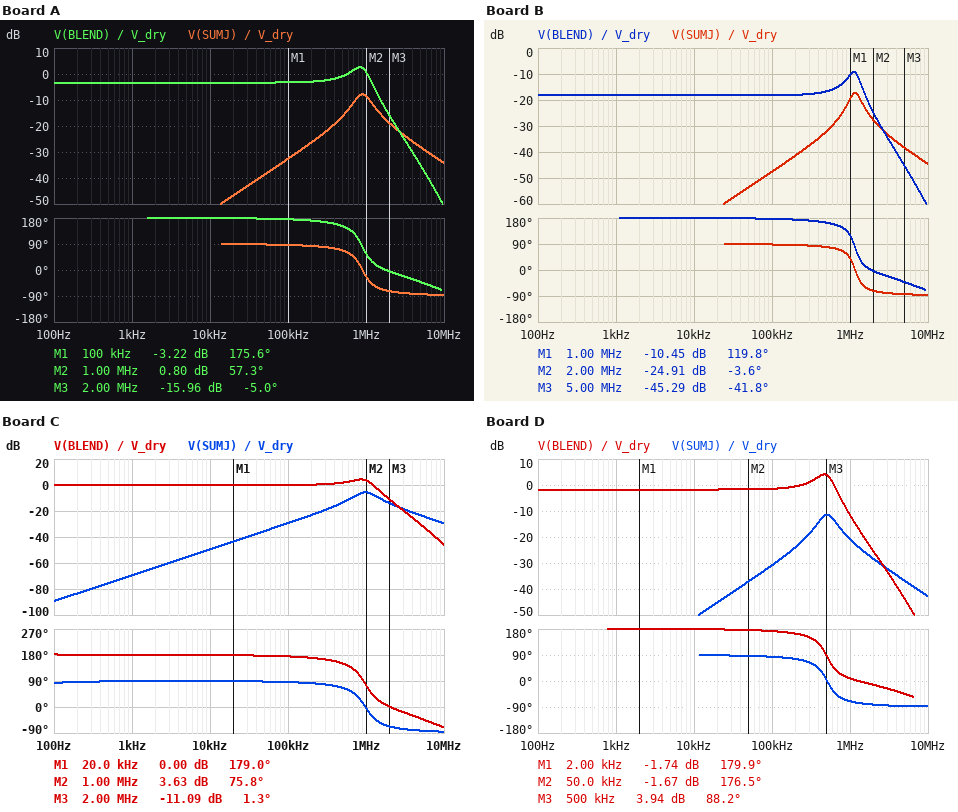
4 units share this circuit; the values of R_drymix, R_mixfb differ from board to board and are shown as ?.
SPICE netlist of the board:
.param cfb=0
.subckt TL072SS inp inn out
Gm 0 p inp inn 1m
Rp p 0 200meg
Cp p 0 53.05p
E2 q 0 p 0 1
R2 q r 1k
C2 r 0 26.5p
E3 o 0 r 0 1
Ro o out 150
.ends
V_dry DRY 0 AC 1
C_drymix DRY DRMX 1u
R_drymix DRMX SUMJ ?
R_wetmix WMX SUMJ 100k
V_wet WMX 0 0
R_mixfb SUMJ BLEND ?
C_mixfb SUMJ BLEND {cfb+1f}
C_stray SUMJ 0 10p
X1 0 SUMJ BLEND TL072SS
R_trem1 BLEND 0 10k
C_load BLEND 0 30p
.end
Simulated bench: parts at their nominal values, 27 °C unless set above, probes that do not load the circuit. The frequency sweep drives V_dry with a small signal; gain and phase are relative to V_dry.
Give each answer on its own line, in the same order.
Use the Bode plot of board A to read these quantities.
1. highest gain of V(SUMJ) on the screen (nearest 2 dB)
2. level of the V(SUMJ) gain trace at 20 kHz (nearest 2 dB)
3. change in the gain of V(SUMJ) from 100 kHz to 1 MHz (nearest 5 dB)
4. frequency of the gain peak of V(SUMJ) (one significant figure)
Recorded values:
-8 dB
-46 dB
25 dB
900 kHz
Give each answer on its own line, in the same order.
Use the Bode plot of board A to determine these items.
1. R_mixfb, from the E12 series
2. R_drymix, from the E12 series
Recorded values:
56 kΩ
82 kΩ
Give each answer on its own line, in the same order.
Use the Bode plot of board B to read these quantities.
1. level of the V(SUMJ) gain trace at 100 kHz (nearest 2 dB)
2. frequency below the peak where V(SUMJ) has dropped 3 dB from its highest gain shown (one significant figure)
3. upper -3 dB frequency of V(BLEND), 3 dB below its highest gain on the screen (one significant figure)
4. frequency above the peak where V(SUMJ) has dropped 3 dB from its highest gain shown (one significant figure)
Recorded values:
-48 dB
1 MHz
1 MHz
1 MHz
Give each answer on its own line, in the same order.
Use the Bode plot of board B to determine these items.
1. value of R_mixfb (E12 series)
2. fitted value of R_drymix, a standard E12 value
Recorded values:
33 kΩ
270 kΩ
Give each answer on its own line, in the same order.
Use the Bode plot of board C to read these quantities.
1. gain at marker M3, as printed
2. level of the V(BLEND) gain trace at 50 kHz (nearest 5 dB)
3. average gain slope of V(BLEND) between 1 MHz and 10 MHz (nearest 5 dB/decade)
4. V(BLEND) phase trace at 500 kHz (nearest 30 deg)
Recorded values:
-11.09 dB
0 dB
-50 dB/decade
150 deg
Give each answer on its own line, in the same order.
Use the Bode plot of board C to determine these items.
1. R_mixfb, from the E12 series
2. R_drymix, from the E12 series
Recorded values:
47 kΩ
47 kΩ
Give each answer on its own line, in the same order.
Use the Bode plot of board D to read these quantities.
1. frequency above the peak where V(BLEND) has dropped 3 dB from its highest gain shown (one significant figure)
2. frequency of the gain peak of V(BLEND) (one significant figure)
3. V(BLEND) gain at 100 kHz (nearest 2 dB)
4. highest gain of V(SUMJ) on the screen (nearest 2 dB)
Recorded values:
600 kHz
500 kHz
-2 dB
-12 dB
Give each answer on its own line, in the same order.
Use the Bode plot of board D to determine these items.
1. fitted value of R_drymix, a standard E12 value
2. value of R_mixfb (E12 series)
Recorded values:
220 kΩ
180 kΩ
